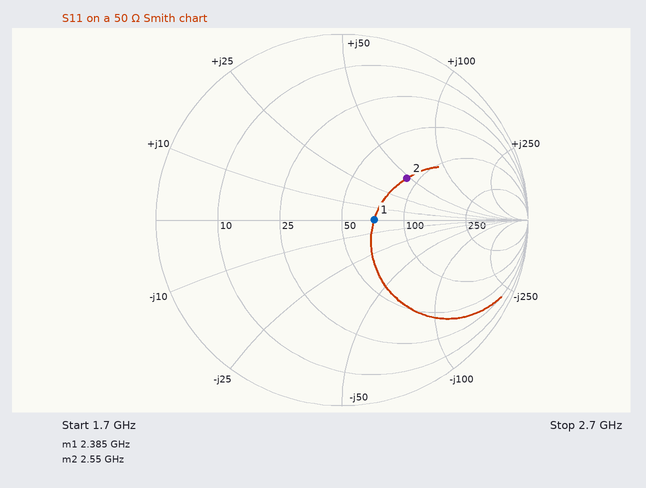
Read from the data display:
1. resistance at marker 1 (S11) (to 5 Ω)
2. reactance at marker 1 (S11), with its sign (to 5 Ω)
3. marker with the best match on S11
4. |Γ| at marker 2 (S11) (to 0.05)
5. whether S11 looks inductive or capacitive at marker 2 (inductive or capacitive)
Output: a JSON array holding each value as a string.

["70 Ω", "0 Ω", "marker 1", "0.40", "inductive"]
